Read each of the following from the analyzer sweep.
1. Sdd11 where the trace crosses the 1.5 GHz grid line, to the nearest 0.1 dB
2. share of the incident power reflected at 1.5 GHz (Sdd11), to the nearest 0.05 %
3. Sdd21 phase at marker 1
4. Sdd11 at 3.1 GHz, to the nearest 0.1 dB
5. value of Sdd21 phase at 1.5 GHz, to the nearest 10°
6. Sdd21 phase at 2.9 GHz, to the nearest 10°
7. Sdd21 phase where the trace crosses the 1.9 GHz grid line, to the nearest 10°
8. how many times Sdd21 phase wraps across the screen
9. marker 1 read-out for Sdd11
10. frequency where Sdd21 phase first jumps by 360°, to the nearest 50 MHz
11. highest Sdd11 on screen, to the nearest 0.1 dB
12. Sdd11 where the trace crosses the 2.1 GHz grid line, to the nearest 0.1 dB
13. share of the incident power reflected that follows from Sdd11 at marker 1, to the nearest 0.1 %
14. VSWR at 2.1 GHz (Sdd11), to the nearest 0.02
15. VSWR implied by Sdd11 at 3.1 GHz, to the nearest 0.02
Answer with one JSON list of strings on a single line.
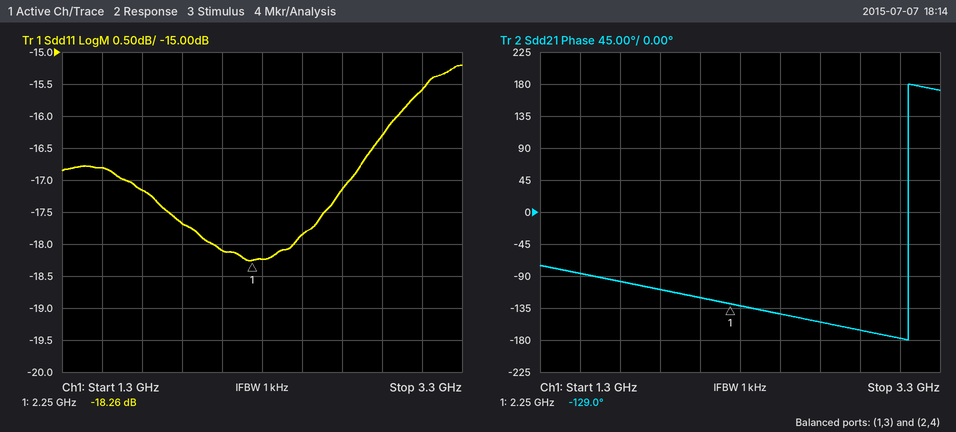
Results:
["-16.8 dB", "2.10 %", "-129.0°", "-15.6 dB", "-90°", "-170°", "-110°", "1", "-18.26 dB", "3.15 GHz", "-15.2 dB", "-18.1 dB", "1.5 %", "1.28", "1.40"]
